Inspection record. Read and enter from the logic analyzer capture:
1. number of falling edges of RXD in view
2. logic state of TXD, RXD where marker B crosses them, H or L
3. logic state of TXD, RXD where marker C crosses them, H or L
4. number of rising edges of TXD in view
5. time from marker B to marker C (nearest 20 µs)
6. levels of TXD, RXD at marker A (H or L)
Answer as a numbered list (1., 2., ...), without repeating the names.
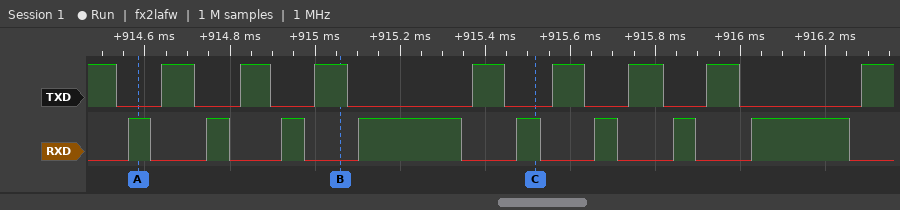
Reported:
1. 8
2. TXD=H, RXD=L
3. TXD=L, RXD=H
4. 8
5. 460 µs
6. TXD=L, RXD=H
